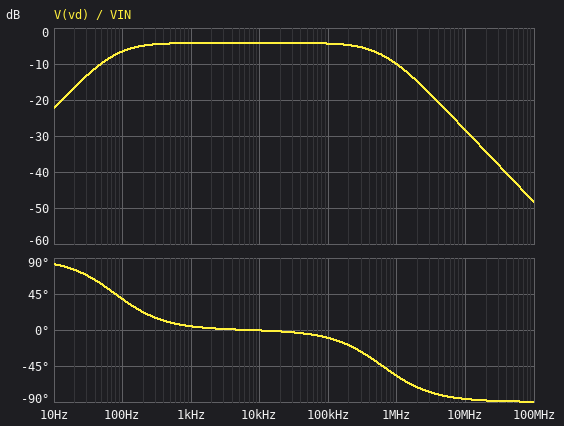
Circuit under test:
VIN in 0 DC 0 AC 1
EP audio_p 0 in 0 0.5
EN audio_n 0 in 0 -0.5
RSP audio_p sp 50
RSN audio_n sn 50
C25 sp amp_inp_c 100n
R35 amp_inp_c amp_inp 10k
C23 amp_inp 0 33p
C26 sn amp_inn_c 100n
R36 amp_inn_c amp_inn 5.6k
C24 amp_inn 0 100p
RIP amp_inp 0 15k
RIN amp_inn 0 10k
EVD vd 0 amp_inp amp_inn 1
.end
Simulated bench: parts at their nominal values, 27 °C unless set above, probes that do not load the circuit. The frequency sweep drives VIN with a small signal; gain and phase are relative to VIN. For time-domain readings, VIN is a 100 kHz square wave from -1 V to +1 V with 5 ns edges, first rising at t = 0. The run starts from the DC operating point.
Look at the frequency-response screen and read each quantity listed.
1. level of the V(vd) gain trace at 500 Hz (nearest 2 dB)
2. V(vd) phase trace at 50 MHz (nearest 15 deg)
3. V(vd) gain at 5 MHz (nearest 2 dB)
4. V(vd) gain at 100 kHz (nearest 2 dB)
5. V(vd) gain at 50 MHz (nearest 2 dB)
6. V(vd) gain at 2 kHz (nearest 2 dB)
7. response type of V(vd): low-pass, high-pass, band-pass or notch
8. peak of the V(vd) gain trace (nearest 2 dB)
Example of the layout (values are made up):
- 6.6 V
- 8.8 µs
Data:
- -4 dB
- -90 deg
- -22 dB
- -4 dB
- -42 dB
- -4 dB
- band-pass
- -4 dB
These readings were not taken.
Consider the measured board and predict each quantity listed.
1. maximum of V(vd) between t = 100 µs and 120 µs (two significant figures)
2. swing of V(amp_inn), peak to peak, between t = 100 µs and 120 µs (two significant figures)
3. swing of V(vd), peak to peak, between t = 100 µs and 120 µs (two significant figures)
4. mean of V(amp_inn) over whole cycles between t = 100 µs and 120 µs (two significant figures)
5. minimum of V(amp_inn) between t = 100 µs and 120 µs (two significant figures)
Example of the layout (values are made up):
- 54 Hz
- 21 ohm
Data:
- 1.2 V
- 640 mV
- 1.2 V
- -300 mV
- -620 mV
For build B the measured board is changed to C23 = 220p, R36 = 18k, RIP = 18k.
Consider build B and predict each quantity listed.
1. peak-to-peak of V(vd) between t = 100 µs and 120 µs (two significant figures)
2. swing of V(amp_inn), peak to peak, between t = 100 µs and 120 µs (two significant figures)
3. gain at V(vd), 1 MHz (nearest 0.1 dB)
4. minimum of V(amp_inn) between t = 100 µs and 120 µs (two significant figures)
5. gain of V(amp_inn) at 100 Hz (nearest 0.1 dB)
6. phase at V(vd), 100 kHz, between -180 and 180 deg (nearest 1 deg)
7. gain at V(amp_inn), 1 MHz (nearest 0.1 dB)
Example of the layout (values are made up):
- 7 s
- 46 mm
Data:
- 960 mV
- 360 mV
- -22.1 dB
- -350 mV
- -16.2 dB
- -34 deg
- -27.4 dB
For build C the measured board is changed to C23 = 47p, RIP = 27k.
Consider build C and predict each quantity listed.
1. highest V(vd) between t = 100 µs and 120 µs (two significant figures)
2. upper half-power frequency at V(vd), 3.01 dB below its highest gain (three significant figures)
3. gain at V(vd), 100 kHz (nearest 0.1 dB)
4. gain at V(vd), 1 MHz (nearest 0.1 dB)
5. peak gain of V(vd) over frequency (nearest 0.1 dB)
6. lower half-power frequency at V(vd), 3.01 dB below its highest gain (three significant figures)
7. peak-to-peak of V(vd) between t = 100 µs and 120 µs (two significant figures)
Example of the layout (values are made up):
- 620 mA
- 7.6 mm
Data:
- 1.3 V
- 452 kHz
- -3.5 dB
- -11.0 dB
- -3.3 dB
- 70.6 Hz
- 1.4 V
